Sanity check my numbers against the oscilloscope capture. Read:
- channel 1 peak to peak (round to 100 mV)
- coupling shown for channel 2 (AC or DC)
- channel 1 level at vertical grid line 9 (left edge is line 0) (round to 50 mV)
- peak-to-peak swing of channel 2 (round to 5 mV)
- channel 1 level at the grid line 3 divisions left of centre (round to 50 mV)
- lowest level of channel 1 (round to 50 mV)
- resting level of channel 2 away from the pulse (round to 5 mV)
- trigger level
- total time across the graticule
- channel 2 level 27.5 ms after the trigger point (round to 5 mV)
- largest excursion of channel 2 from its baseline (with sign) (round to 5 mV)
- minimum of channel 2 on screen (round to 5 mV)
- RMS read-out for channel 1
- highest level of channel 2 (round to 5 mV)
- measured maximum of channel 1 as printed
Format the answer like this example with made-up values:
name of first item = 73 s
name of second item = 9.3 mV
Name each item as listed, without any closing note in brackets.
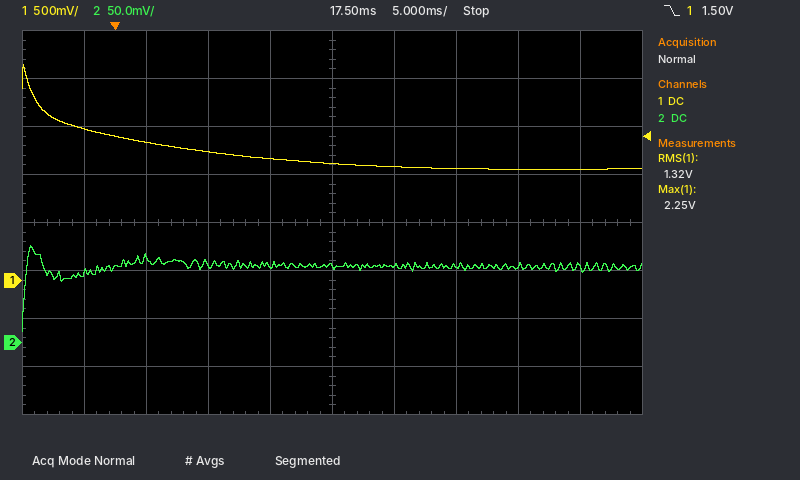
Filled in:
channel 1 peak to peak = 1.10 V
coupling shown for channel 2 = DC
channel 1 level at vertical grid line 9 (left edge is line 0) = 1.15 V
peak-to-peak swing of channel 2 = 90 mV
channel 1 level at the grid line 3 divisions left of centre = 1.45 V
lowest level of channel 1 = 1.15 V
resting level of channel 2 away from the pulse = 80 mV
trigger level = 1.50 V
total time across the graticule = 50 ms
channel 2 level 27.5 ms after the trigger point = 80 mV
largest excursion of channel 2 from its baseline (with sign) = -70 mV
minimum of channel 2 on screen = 10 mV
RMS read-out for channel 1 = 1.32 V
highest level of channel 2 = 100 mV
measured maximum of channel 1 as printed = 2.25 V
